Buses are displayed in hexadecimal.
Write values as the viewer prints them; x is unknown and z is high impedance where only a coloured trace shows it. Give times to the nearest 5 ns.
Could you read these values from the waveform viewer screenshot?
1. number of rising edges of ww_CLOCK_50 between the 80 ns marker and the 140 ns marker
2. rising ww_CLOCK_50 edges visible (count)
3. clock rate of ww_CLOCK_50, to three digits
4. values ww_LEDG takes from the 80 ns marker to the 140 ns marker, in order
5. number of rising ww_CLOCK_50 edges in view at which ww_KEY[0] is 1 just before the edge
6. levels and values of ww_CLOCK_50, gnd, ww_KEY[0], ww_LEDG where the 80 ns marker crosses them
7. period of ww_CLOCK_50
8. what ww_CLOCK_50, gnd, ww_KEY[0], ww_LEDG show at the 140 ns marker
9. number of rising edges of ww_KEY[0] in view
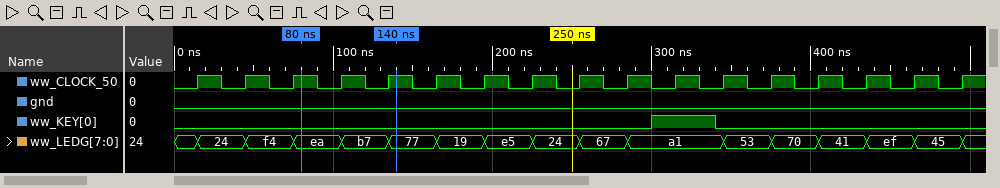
2
17
33.3 MHz
ea, b7, 77
1
ww_CLOCK_50=1, gnd=0, ww_KEY[0]=0, ww_LEDG=ea
30 ns
ww_CLOCK_50=1, gnd=0, ww_KEY[0]=0, ww_LEDG=77
1
